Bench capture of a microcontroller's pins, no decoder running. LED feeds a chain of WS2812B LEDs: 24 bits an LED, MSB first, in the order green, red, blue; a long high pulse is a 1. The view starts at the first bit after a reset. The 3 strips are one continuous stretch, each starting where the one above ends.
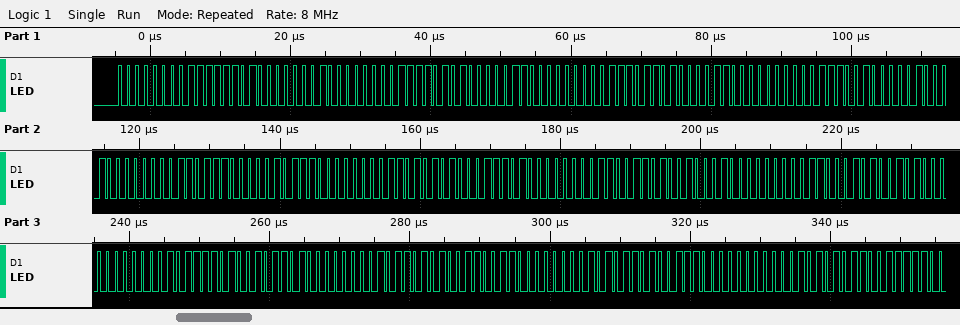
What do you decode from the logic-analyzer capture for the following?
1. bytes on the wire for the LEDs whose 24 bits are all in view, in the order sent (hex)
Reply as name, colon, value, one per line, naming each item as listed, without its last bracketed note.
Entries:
bytes on the wire for the LEDs whose 24 bits are all in view, in the order sent: 00 FD 01 00 F5 06 00 ED 0C 00 E4 11 00 DC 17 00 D5 1D 00 CD 22 00 C5 28 00 BD 2D 00 B5 33 00 AD 38 00 AB 3E
